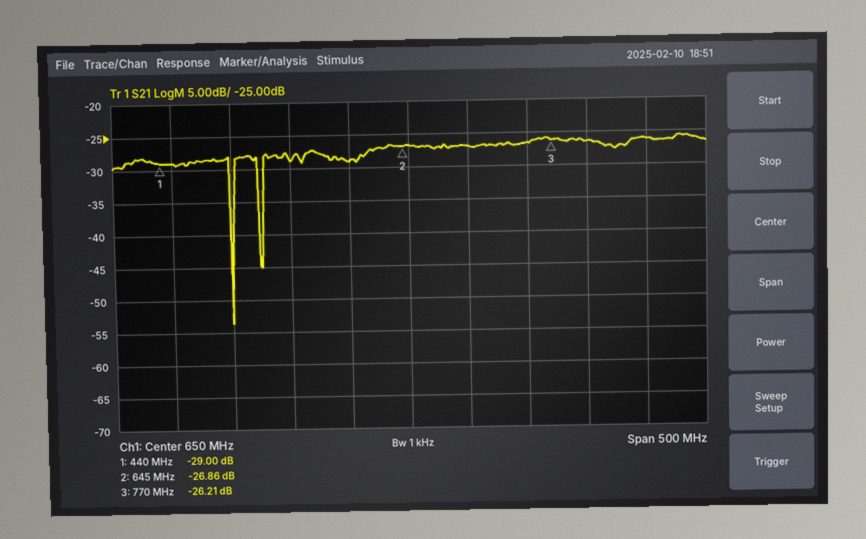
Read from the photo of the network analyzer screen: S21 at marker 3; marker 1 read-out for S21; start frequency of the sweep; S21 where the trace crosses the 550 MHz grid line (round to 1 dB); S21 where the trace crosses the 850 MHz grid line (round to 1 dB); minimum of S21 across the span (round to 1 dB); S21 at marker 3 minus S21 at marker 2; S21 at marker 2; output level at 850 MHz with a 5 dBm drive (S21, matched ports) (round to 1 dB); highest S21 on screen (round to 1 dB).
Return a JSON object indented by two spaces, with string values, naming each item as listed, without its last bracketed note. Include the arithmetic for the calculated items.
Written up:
{
  "S21 at marker 3": "-26.21 dB",
  "marker 1 read-out for S21": "-29.00 dB",
  "start frequency of the sweep": "400 MHz",
  "S21 where the trace crosses the 550 MHz grid line": "-29 dB",
  "S21 where the trace crosses the 850 MHz grid line": "-26 dB",
  "minimum of S21 across the span": "-54 dB",
  "S21 at marker 3 minus S21 at marker 2": "-26.21 − (-26.86) = 0.65 dB",
  "S21 at marker 2": "-26.86 dB",
  "output level at 850 MHz with a 5 dBm drive (S21, matched ports)": "5 dBm + (-26 dB) = -21 dBm",
  "highest S21 on screen": "-26 dB"
}
